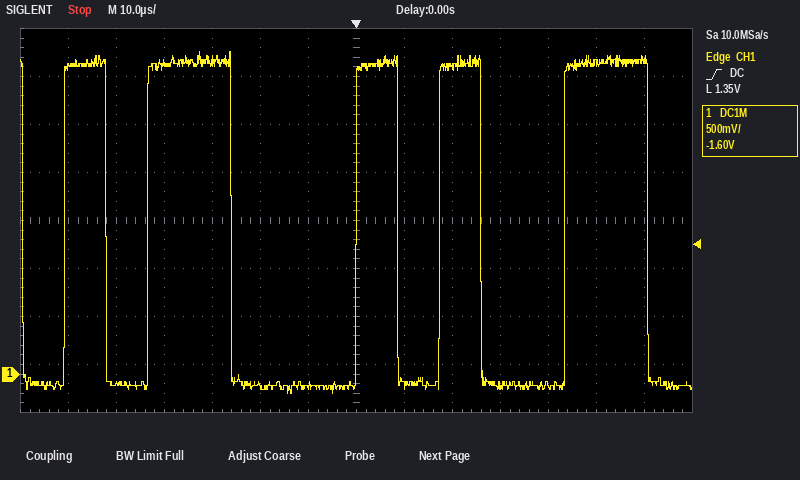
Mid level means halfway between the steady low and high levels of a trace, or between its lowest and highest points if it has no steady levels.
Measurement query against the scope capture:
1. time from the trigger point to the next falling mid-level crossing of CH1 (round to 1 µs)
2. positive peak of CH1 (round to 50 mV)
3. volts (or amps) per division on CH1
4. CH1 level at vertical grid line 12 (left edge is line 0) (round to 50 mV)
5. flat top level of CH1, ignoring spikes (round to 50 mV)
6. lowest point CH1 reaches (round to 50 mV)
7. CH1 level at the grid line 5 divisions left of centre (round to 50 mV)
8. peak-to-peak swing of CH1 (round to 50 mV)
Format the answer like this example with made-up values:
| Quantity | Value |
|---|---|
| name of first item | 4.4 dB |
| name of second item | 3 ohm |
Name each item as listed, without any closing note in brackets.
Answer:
| Quantity | Value |
|---|---|
| time from the trigger point to the next falling mid-level crossing of CH1 | 9 µs |
| positive peak of CH1 | 3.35 V |
| volts (or amps) per division on CH1 | 500 mV |
| CH1 level at vertical grid line 12 (left edge is line 0) | 3.25 V |
| flat top level of CH1, ignoring spikes | 3.25 V |
| lowest point CH1 reaches | -200 mV |
| CH1 level at the grid line 5 divisions left of centre | -100 mV |
| peak-to-peak swing of CH1 | 3.55 V |
